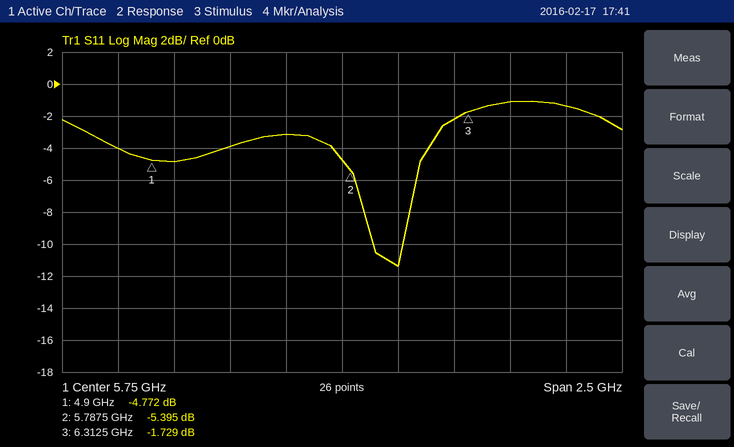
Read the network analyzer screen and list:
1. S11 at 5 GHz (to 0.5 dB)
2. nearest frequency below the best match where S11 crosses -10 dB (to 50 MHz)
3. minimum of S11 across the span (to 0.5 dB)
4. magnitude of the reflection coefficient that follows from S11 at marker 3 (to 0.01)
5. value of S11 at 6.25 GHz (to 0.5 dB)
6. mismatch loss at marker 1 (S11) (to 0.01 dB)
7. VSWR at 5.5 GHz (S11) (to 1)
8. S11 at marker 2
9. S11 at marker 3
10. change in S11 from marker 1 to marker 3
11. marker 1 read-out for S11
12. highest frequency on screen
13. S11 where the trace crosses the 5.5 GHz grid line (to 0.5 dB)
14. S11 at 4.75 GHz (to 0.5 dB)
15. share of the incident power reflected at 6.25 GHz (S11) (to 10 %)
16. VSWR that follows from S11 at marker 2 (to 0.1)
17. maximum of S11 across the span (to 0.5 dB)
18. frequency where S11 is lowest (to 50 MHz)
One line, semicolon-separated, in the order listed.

-5.0 dB; 5.90 GHz; -11.5 dB; 0.82; -2.0 dB; 1.76 dB; 6; -5.395 dB; -1.729 dB; 3.043 dB; -4.772 dB; 7 GHz; -3.0 dB; -4.0 dB; 60 %; 3.3; -1.0 dB; 6.00 GHz
